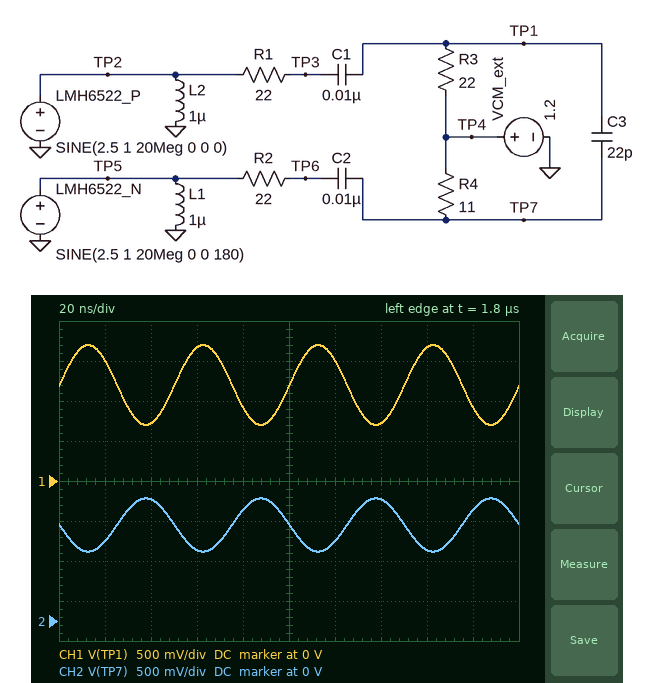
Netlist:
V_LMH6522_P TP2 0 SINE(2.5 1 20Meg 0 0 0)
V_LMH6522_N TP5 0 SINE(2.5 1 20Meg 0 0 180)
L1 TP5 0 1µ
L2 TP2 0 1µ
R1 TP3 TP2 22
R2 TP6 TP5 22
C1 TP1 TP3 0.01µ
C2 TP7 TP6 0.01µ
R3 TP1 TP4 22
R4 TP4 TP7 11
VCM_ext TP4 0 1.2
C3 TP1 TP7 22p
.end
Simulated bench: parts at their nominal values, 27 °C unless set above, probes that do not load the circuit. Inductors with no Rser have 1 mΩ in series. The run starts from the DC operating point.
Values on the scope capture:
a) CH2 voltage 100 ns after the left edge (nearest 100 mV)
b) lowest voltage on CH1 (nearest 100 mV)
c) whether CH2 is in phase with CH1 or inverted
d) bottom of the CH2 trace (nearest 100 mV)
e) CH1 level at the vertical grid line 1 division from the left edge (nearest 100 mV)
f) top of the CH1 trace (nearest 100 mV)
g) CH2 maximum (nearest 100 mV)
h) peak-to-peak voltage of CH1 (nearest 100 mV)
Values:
1.2 V
700 mV
inverted
900 mV
1.5 V
1.7 V
1.5 V
1.0 V
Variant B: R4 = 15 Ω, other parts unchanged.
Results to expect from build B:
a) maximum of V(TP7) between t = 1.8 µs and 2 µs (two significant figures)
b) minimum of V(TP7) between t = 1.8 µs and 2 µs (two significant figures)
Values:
1.6 V
800 mV
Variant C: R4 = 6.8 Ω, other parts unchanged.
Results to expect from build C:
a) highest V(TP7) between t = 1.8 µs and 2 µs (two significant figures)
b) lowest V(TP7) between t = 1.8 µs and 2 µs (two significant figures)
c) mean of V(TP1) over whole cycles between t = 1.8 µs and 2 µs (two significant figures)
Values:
1.4 V
960 mV
1.2 V
